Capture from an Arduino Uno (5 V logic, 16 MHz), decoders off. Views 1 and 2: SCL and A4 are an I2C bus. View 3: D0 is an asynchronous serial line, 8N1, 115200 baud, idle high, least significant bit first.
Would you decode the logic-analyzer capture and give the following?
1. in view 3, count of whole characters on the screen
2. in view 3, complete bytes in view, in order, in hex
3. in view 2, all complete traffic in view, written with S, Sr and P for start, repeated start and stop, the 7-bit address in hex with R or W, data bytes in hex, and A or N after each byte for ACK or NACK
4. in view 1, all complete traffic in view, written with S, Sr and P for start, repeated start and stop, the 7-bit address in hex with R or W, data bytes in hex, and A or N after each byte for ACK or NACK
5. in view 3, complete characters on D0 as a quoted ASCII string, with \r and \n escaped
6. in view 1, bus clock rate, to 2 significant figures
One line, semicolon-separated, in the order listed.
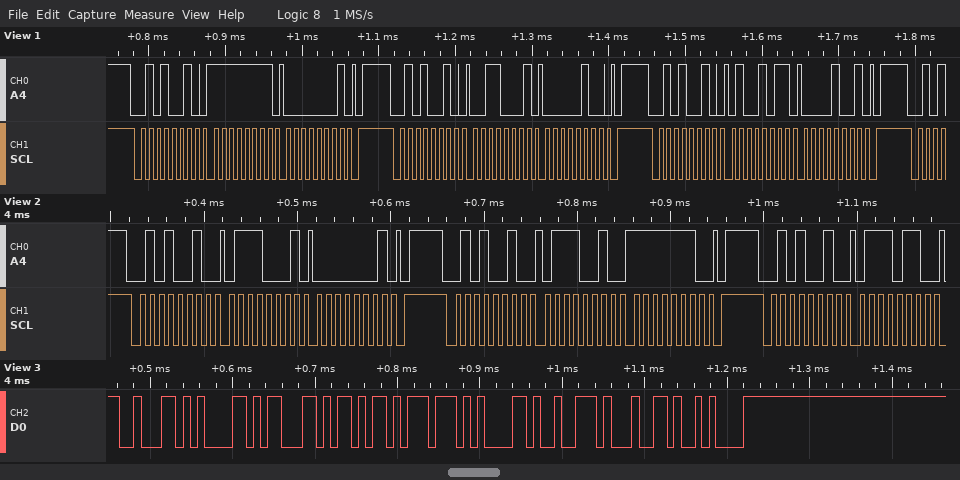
9; 62 61 63 6B 77 61 72 64 0A; S 29W A 71 A 01 A P S 29W A 72 A FE A P S 29W A 76 A; S 29W A FF A 01 A P S 29W A 31 A 04 A P S 29W A 4B A 09 A P; "backward\n"; 100 kHz
